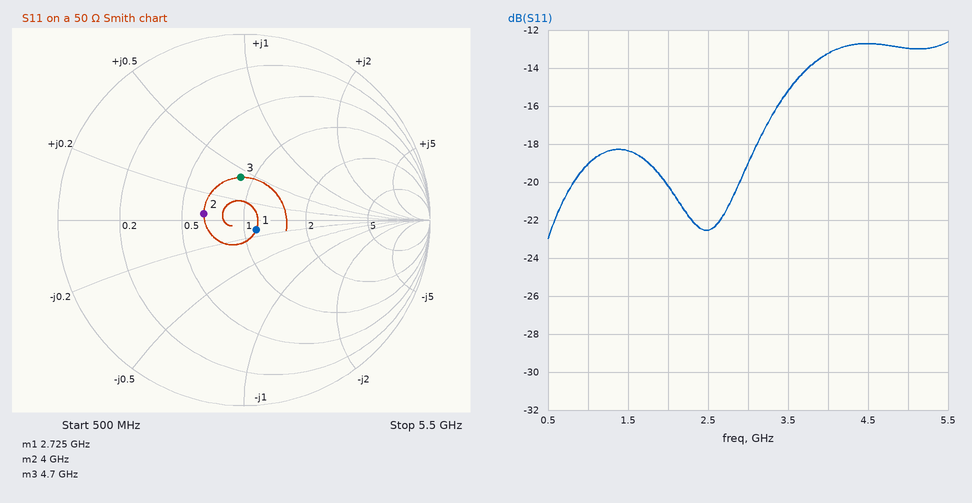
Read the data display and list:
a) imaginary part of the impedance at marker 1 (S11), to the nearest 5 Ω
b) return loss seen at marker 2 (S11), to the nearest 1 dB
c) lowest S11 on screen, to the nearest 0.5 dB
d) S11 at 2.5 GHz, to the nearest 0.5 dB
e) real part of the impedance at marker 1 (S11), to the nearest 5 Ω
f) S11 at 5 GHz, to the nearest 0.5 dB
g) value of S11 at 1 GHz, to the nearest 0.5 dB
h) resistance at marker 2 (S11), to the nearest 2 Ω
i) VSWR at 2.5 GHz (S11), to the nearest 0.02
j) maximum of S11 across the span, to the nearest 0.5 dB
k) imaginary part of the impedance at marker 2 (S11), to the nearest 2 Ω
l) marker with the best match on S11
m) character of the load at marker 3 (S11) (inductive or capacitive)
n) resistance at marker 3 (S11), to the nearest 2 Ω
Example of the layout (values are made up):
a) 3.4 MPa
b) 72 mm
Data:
a) -5 Ω
b) 13 dB
c) -23.0 dB
d) -22.5 dB
e) 55 Ω
f) -13.0 dB
g) -19.0 dB
h) 32 Ω
i) 1.16
j) -12.5 dB
k) +2 Ω
l) marker 1
m) inductive
n) 44 Ω
